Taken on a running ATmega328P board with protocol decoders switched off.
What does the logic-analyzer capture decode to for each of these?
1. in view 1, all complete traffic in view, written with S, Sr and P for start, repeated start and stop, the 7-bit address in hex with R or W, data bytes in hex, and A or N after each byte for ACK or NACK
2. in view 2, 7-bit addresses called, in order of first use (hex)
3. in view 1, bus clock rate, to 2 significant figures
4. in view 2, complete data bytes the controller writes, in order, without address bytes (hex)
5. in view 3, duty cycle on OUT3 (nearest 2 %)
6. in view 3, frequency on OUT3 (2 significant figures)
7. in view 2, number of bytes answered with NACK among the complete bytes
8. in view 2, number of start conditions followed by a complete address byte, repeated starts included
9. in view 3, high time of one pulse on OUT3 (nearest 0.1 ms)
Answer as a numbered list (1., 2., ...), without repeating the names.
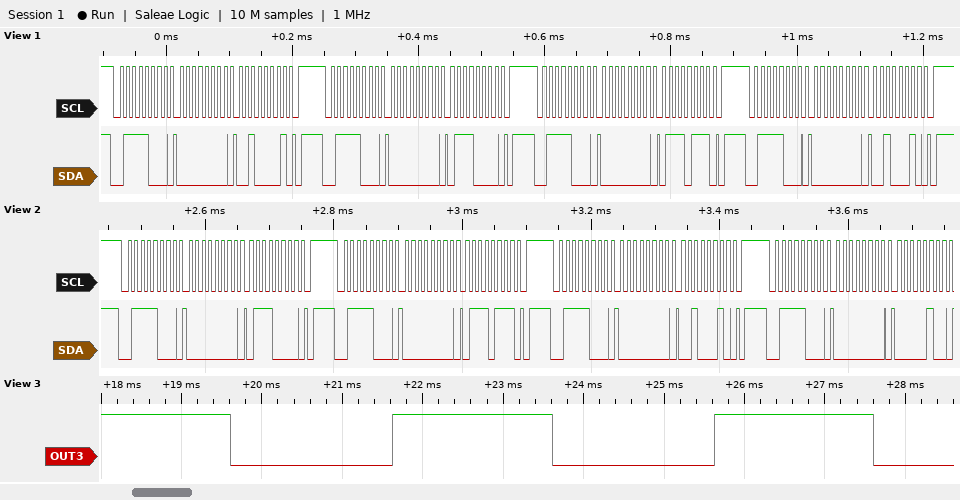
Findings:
1. S 3CW A 00 A 21 A P S 3CW A 00 A 70 A P S 3CW A 00 A 77 A P S 3CW A 00 A 22 A P
2. 0x3C
3. 100 kHz
4. 00 70 00 77 00 22 00 04
5. 50 %
6. 250 Hz
7. 0
8. 4
9. 2.0 ms
